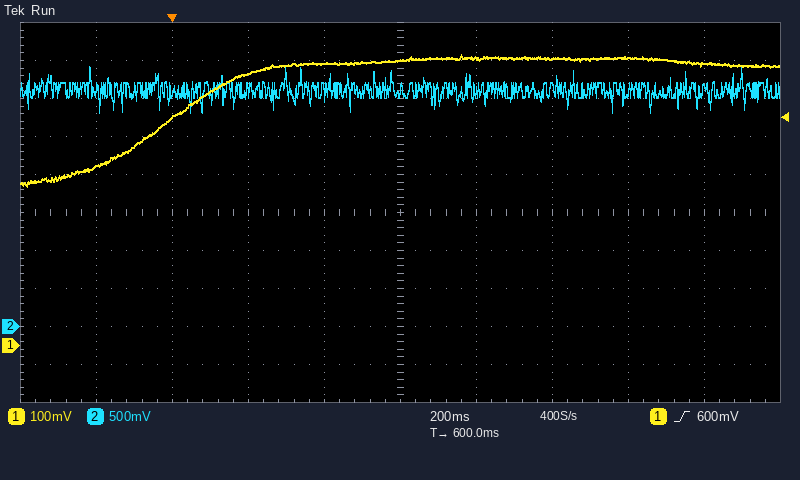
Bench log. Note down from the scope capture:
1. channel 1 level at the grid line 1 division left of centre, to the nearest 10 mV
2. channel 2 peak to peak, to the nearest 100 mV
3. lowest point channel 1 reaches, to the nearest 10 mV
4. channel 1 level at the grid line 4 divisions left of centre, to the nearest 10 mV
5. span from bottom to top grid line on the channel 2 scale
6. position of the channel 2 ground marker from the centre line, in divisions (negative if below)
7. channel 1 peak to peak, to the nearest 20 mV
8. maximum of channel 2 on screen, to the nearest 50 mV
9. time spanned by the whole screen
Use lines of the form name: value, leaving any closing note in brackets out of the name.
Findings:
channel 1 level at the grid line 1 division left of centre, to the nearest 10 mV: 740 mV
channel 2 peak to peak, to the nearest 100 mV: 600 mV
lowest point channel 1 reaches, to the nearest 10 mV: 420 mV
channel 1 level at the grid line 4 divisions left of centre, to the nearest 10 mV: 470 mV
span from bottom to top grid line on the channel 2 scale: 5 V
position of the channel 2 ground marker from the centre line, in divisions: -3.0 div
channel 1 peak to peak, to the nearest 20 mV: 340 mV
maximum of channel 2 on screen, to the nearest 50 mV: 3.40 V
time spanned by the whole screen: 2 s
